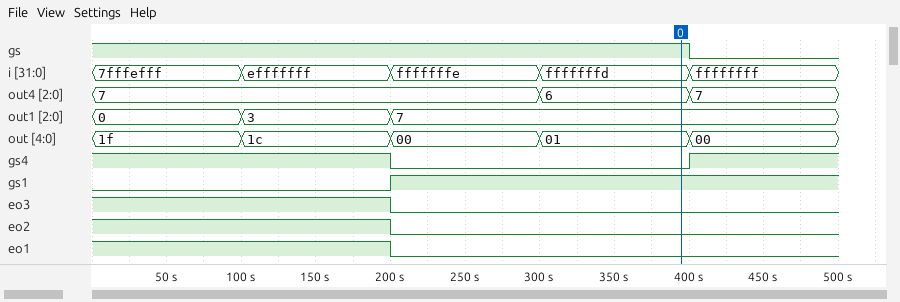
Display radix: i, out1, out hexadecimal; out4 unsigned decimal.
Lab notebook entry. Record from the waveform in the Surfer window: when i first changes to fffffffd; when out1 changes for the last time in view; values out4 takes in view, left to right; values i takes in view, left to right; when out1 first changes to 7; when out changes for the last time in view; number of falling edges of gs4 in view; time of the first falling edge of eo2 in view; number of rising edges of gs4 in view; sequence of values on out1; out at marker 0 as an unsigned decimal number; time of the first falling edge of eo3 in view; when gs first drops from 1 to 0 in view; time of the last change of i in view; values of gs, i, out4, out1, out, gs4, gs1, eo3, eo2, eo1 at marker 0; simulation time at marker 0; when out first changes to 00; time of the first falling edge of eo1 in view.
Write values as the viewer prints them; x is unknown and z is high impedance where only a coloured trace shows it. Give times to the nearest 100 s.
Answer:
300 s
200 s
7, 6, 7
7fffefff, efffffff, fffffffe, fffffffd, ffffffff
200 s
400 s
1
200 s
1
0, 3, 7
1
200 s
400 s
400 s
gs=1, i=fffffffd, out4=6, out1=7, out=01, gs4=0, gs1=1, eo3=0, eo2=0, eo1=0
400 s
200 s
200 s
